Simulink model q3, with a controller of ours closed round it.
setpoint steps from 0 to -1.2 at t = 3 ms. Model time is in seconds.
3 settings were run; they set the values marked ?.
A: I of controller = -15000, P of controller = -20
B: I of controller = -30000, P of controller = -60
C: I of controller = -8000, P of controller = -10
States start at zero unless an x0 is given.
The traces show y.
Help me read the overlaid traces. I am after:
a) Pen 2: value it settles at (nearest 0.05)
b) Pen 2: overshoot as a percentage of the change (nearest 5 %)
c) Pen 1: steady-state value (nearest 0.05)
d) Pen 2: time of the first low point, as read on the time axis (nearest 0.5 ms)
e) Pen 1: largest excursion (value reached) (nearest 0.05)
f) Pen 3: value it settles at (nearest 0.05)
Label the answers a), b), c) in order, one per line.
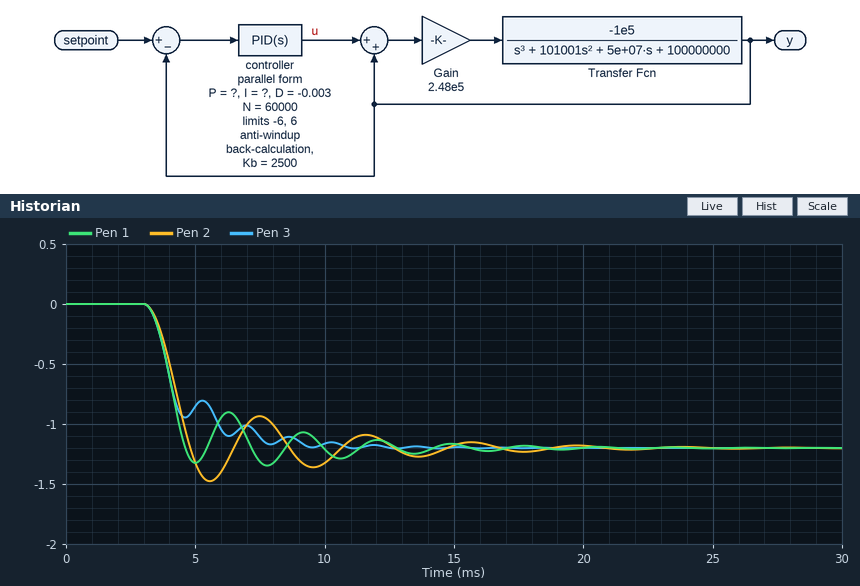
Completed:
a) -1.20
b) 25 %
c) -1.20
d) 5.5 ms
e) -1.35
f) -1.20
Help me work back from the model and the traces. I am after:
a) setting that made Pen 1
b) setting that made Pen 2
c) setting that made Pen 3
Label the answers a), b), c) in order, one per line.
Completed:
a) A
b) C
c) B
